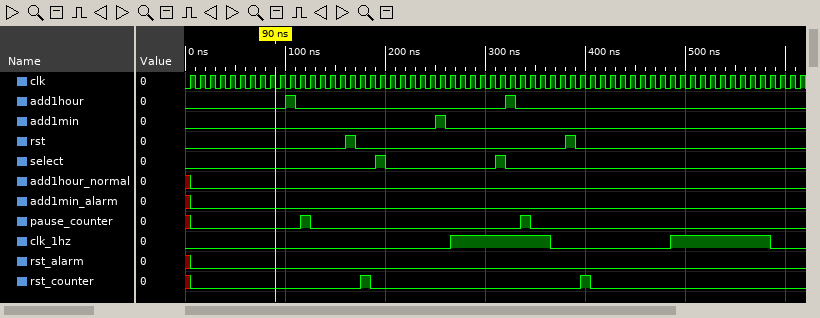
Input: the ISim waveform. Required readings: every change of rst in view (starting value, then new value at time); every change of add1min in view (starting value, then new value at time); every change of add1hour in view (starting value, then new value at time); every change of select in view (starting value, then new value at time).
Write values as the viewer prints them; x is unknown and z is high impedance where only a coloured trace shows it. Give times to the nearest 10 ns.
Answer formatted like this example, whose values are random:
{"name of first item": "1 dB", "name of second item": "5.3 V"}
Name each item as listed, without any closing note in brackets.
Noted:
{"every change of rst in view": "0, 1 at 160 ns, 0 at 170 ns, 1 at 380 ns, 0 at 390 ns", "every change of add1min in view": "0, 1 at 250 ns, 0 at 260 ns", "every change of add1hour in view": "0, 1 at 100 ns, 0 at 110 ns, 1 at 320 ns, 0 at 330 ns", "every change of select in view": "0, 1 at 190 ns, 0 at 200 ns, 1 at 310 ns, 0 at 320 ns"}
